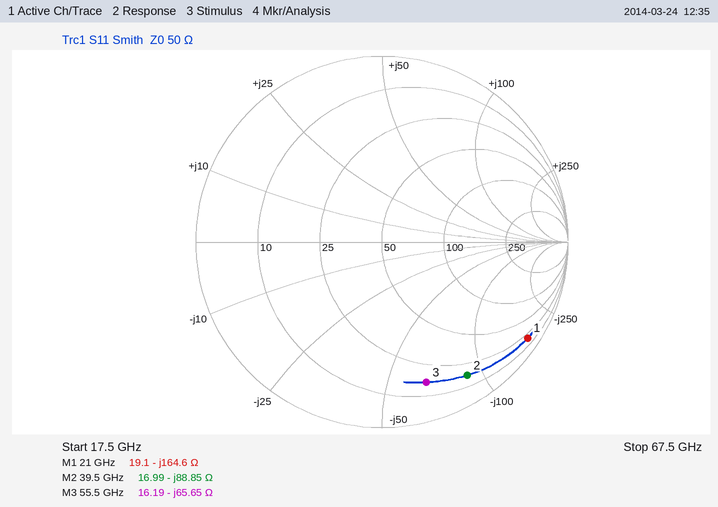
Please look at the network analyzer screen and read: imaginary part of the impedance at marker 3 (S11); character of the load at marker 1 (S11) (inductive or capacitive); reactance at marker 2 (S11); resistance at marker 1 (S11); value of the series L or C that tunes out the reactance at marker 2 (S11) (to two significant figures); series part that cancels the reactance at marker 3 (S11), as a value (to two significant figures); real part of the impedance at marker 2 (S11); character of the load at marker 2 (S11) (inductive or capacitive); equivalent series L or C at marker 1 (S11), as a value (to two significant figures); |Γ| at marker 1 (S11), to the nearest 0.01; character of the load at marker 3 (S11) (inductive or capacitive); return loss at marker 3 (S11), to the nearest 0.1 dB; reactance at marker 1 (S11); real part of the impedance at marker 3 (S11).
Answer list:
-65.65 Ω
capacitive
-88.85 Ω
19.1 Ω
360 pH
190 pH
16.99 Ω
capacitive
46 fF
0.94
capacitive
2.0 dB
-164.6 Ω
16.19 Ω
